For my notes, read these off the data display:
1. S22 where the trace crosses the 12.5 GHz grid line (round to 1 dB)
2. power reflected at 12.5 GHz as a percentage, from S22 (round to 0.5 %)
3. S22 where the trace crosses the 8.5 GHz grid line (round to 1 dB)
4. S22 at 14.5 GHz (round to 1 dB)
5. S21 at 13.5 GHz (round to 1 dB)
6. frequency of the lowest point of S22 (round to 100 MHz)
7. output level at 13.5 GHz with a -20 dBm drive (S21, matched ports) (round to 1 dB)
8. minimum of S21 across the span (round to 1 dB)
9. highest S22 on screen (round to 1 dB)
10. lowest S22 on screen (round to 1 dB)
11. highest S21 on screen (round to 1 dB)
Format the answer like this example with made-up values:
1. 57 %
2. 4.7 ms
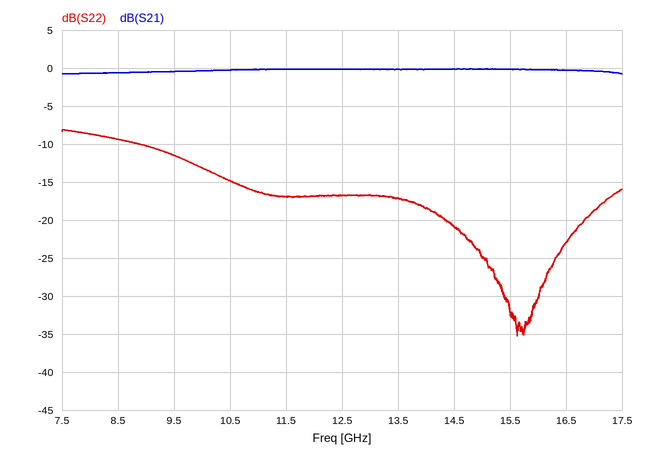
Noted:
1. -17 dB
2. 2.0 %
3. -9 dB
4. -21 dB
5. 0 dB
6. 15.6 GHz
7. -20 dBm
8. -1 dB
9. -8 dB
10. -35 dB
11. 0 dB
